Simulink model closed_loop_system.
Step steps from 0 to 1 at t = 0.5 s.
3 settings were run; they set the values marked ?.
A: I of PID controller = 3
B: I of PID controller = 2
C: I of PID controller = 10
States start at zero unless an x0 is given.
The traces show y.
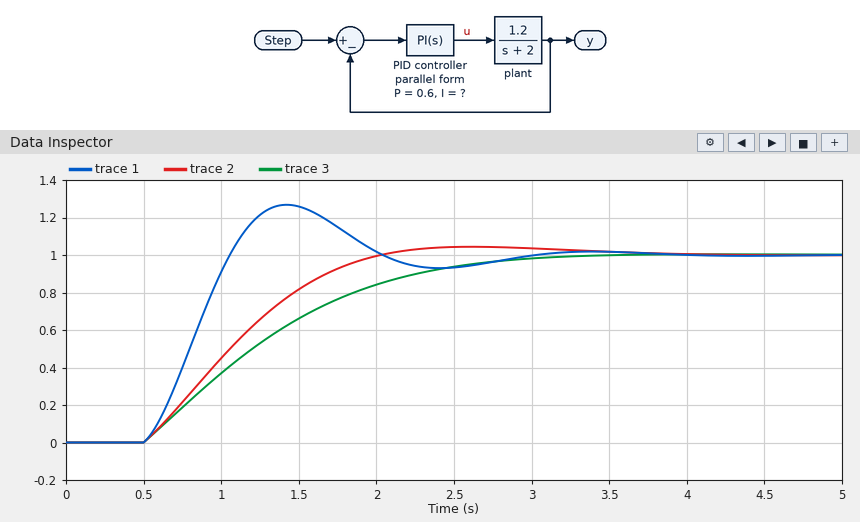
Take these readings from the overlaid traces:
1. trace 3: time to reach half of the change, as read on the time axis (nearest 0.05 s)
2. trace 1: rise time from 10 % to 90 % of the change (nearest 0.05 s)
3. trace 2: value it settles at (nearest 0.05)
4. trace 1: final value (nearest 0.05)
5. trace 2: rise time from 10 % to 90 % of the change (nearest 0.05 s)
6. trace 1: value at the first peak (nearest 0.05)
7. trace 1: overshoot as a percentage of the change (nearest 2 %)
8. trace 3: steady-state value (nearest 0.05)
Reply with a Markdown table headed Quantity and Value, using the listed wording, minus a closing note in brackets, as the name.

| Quantity | Value |
|---|---|
| trace 3: time to reach half of the change, as read on the time axis | 1.20 s |
| trace 1: rise time from 10 % to 90 % of the change | 0.40 s |
| trace 2: value it settles at | 1.00 |
| trace 1: final value | 1.00 |
| trace 2: rise time from 10 % to 90 % of the change | 1.05 s |
| trace 1: value at the first peak | 1.25 |
| trace 1: overshoot as a percentage of the change | 26 % |
| trace 3: steady-state value | 1.00 |
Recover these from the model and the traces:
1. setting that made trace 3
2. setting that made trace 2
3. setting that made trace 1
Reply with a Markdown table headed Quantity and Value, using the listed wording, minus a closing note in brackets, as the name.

| Quantity | Value |
|---|---|
| setting that made trace 3 | B |
| setting that made trace 2 | A |
| setting that made trace 1 | C |
